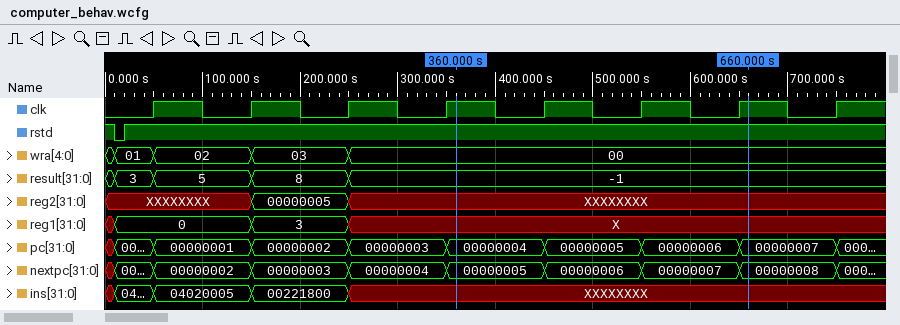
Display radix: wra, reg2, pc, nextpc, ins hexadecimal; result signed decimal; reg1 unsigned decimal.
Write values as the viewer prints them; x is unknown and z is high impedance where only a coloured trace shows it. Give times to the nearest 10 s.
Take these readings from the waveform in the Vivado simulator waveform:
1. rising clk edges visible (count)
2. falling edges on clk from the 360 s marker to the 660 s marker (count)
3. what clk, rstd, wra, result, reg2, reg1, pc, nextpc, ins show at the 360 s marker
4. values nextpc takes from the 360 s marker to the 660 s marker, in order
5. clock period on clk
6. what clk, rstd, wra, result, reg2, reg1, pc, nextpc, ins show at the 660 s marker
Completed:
8
3
clk=1, rstd=1, wra=00, result=-1, reg2=XXXXXXXX, reg1=X, pc=00000004, nextpc=00000005, ins=XXXXXXXX
00000005, 00000006, 00000007, 00000008
100 s
clk=1, rstd=1, wra=00, result=-1, reg2=XXXXXXXX, reg1=X, pc=00000007, nextpc=00000008, ins=XXXXXXXX
